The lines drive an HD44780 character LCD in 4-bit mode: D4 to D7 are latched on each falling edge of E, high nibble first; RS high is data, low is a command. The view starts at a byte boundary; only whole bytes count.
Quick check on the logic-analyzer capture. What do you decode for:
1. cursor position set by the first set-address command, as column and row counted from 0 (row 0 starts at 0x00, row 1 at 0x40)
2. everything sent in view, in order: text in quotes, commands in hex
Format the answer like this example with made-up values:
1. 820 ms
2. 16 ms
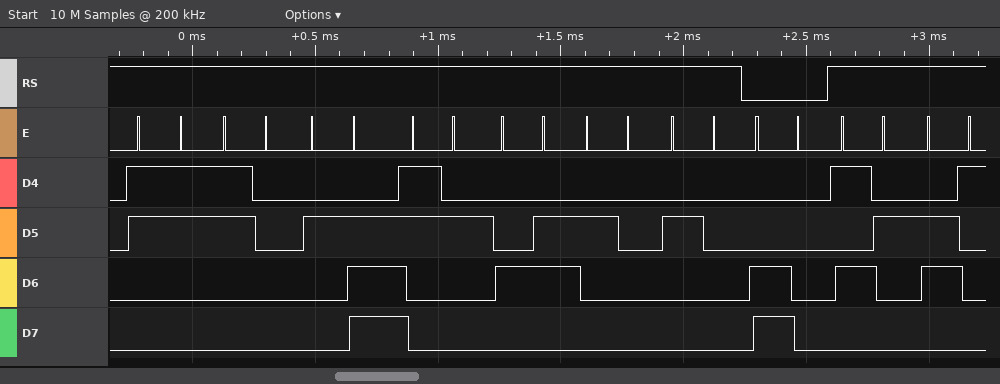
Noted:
1. column 0, row 1
2. "30.2F  " 0xC0 "Ra"
